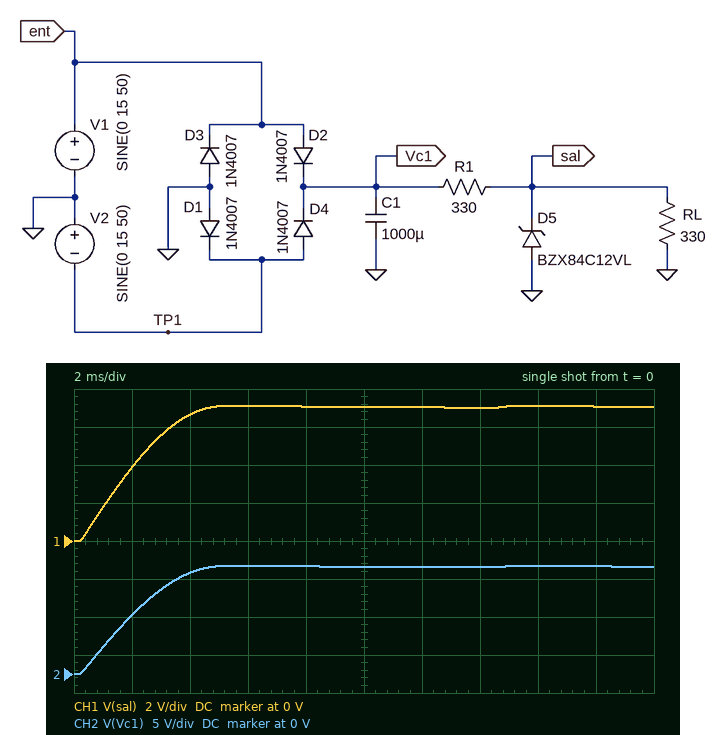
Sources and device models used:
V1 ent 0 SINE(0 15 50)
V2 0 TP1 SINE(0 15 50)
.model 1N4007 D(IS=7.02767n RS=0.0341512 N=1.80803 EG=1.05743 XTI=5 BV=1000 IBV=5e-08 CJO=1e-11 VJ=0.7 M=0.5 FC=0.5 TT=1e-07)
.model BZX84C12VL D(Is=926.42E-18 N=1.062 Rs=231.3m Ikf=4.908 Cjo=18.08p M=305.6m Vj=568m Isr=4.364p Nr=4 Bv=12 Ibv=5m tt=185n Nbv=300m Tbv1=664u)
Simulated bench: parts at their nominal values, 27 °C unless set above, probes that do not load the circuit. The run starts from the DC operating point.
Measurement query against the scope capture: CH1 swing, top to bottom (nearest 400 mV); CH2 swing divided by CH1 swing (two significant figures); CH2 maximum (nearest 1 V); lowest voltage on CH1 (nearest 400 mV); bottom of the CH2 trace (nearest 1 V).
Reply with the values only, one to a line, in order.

7.2 V
2.0
14 V
0 V
0 V
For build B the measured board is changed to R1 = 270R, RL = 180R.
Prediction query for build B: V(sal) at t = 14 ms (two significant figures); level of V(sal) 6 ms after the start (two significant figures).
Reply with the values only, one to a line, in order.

5.6 V
5.7 V
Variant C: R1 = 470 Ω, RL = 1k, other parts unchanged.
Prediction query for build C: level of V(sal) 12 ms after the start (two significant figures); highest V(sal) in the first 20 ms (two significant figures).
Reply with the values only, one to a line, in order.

9.6 V
9.7 V
